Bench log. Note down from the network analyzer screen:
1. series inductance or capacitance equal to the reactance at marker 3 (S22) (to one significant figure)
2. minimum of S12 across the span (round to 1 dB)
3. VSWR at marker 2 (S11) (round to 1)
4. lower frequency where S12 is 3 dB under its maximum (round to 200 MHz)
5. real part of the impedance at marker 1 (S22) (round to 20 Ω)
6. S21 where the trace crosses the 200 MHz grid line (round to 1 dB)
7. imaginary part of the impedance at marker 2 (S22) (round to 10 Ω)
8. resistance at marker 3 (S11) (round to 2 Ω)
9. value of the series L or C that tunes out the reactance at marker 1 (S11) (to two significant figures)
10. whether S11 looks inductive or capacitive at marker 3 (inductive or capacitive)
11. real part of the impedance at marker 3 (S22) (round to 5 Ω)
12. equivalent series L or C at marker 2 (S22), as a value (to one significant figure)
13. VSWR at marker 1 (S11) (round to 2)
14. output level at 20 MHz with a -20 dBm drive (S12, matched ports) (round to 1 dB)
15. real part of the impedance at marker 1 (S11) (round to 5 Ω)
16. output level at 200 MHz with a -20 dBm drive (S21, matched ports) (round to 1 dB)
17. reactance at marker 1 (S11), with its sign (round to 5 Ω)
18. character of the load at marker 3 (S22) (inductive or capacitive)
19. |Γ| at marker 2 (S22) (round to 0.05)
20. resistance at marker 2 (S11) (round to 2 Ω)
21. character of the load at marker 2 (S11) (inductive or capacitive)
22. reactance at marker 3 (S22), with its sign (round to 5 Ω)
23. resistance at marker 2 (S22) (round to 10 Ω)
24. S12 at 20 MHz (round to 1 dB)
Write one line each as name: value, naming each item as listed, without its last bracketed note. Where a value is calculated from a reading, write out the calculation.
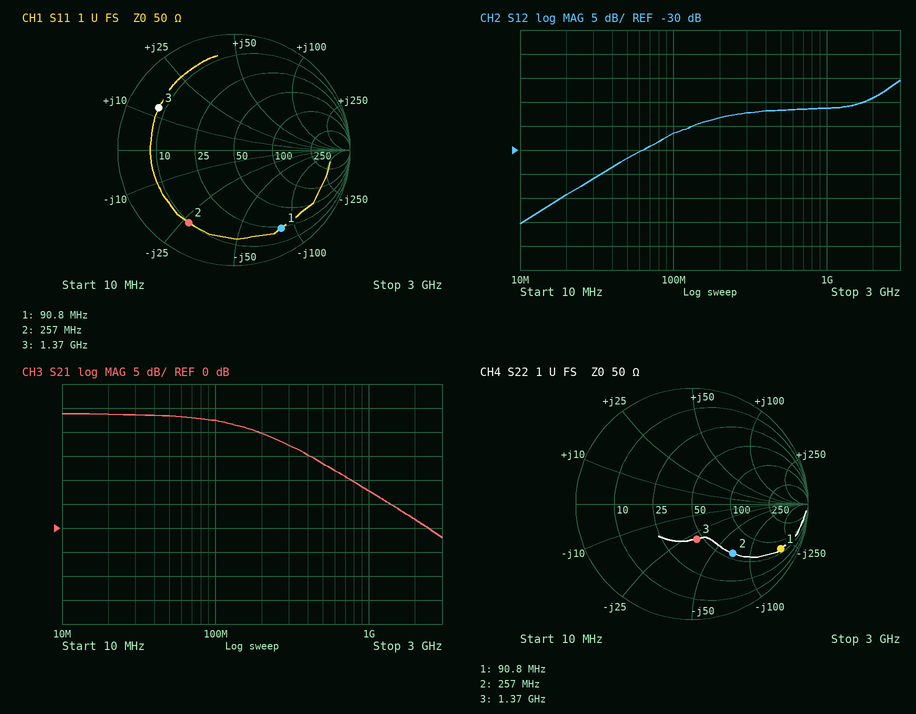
series inductance or capacitance equal to the reactance at marker 3 (S22): C = 1/(2π × 1.37 GHz × 30 Ω) ≈ 4 pF
minimum of S12 across the span: -45 dB
VSWR at marker 2 (S11): 7
lower frequency where S12 is 3 dB under its maximum: 2.2 GHz
real part of the impedance at marker 1 (S22): 60 Ω
S21 where the trace crosses the 200 MHz grid line: 20 dB
imaginary part of the impedance at marker 2 (S22): -70 Ω
resistance at marker 3 (S11): 8 Ω
value of the series L or C that tunes out the reactance at marker 1 (S11): L = 85 Ω/(2π × 90.8 MHz) ≈ 149 nH, so 150 nH to two significant figures
whether S11 looks inductive or capacitive at marker 3: inductive
real part of the impedance at marker 3 (S22): 45 Ω
equivalent series L or C at marker 2 (S22), as a value: C = 1/(2π × 257 MHz × 70 Ω) ≈ 9 pF
VSWR at marker 1 (S11): 8
output level at 20 MHz with a -20 dBm drive (S12, matched ports): -20 dBm + (-39 dB) = -59 dBm
real part of the impedance at marker 1 (S11): 25 Ω
output level at 200 MHz with a -20 dBm drive (S21, matched ports): -20 dBm + (20 dB) = 0 dBm
reactance at marker 1 (S11), with its sign: -85 Ω
character of the load at marker 3 (S22): capacitive
|Γ| at marker 2 (S22): 0.55
resistance at marker 2 (S11): 10 Ω
character of the load at marker 2 (S11): capacitive
reactance at marker 3 (S22), with its sign: -30 Ω
resistance at marker 2 (S22): 60 Ω
S12 at 20 MHz: -39 dB
